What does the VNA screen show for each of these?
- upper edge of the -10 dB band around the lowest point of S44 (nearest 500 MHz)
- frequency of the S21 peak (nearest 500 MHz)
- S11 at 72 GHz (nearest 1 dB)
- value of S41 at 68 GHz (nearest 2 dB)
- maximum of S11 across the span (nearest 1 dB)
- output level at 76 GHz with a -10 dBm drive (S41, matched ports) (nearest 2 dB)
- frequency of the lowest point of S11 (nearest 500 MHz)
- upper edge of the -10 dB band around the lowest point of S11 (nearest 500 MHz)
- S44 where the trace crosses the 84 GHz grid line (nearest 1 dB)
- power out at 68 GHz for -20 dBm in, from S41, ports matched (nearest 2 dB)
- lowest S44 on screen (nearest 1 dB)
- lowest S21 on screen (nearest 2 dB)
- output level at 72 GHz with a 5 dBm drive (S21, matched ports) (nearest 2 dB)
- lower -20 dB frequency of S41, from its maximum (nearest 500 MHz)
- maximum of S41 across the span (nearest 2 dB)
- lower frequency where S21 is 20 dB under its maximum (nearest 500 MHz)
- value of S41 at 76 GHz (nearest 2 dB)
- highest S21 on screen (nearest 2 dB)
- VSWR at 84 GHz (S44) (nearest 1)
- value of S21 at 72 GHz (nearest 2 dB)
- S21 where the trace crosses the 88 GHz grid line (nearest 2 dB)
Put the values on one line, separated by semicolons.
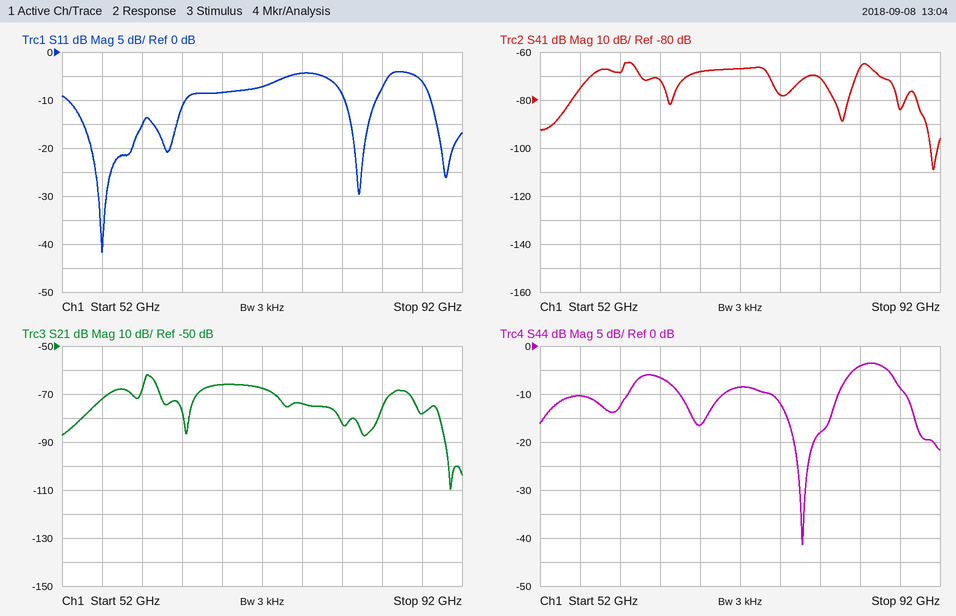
82.0 GHz; 60.5 GHz; -7 dB; -68 dB; -4 dB; -88 dBm; 56.0 GHz; 64.5 GHz; -4 dB; -88 dBm; -41 dB; -110 dB; -62 dBm; 54.5 GHz; -64 dB; 53.5 GHz; -78 dB; -62 dB; 4; -68 dB; -78 dB
